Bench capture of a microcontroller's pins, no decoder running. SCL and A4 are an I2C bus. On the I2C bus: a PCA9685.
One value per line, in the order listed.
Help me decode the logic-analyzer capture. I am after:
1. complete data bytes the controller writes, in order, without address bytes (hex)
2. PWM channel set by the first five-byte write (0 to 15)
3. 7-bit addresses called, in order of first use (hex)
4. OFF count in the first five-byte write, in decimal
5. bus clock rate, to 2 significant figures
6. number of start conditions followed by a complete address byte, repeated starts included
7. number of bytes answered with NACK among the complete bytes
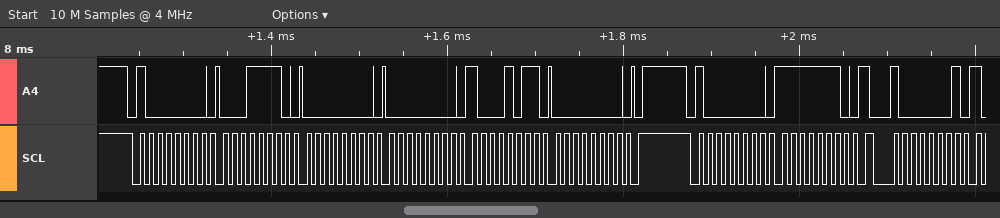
1E 00 00 8B 00 FE
6
0x40
139
100 kHz
3
0
